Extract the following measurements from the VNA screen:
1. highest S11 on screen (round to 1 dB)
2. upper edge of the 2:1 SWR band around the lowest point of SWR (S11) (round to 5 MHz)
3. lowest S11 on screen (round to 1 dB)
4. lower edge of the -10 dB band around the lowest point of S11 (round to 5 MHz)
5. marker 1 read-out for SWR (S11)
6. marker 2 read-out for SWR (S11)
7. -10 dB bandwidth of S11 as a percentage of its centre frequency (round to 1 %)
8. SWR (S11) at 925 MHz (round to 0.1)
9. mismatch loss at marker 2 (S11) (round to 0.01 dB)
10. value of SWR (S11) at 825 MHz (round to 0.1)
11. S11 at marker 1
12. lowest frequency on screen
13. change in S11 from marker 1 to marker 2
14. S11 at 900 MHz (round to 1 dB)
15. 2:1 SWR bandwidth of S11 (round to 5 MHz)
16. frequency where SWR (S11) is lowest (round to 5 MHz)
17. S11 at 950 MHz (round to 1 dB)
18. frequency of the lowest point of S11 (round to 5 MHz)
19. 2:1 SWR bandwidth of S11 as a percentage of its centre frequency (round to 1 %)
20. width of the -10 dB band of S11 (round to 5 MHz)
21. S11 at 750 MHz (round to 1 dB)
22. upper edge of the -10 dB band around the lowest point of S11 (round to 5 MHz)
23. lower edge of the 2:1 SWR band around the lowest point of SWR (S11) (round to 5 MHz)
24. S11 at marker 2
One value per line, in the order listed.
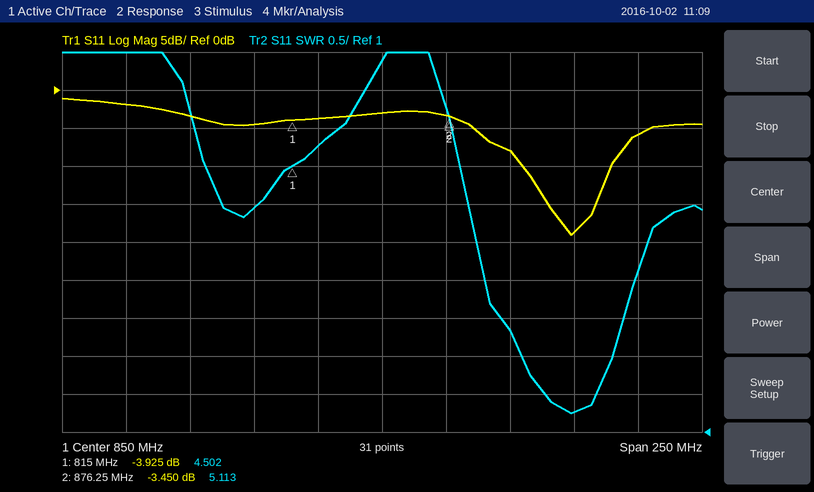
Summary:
-1 dB
940 MHz
-19 dB
905 MHz
4.502
5.113
4 %
1.3
2.61 dB
4.8
-3.925 dB
725 MHz
0.475 dB
-8 dB
35 MHz
925 MHz
-6 dB
925 MHz
4 %
35 MHz
-2 dB
940 MHz
905 MHz
-3.450 dB
